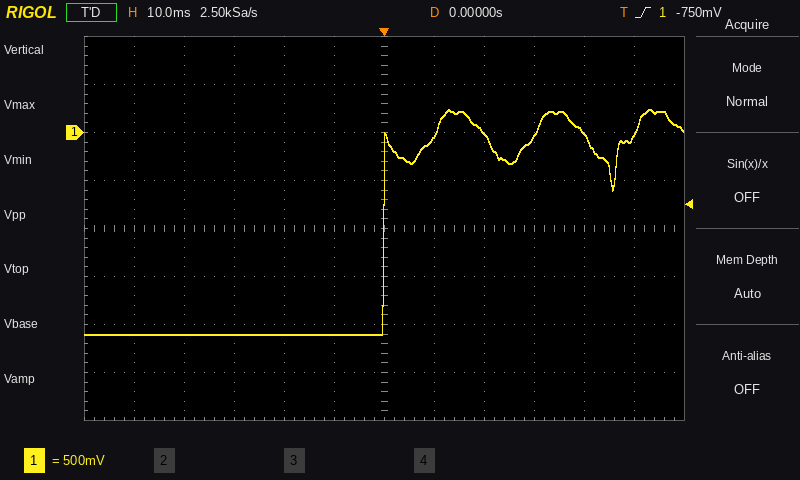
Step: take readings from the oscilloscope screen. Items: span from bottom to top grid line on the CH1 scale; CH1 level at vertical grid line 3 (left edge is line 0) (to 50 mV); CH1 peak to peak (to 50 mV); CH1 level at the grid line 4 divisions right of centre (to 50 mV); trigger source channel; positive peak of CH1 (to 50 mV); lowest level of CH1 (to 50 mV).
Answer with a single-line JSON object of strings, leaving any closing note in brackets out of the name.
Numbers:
{"span from bottom to top grid line on the CH1 scale": "4 V", "CH1 level at vertical grid line 3 (left edge is line 0)": "-2.10 V", "CH1 peak to peak": "2.35 V", "CH1 level at the grid line 4 divisions right of centre": "0 mV", "trigger source channel": "CH1", "positive peak of CH1": "250 mV", "lowest level of CH1": "-2.10 V"}
